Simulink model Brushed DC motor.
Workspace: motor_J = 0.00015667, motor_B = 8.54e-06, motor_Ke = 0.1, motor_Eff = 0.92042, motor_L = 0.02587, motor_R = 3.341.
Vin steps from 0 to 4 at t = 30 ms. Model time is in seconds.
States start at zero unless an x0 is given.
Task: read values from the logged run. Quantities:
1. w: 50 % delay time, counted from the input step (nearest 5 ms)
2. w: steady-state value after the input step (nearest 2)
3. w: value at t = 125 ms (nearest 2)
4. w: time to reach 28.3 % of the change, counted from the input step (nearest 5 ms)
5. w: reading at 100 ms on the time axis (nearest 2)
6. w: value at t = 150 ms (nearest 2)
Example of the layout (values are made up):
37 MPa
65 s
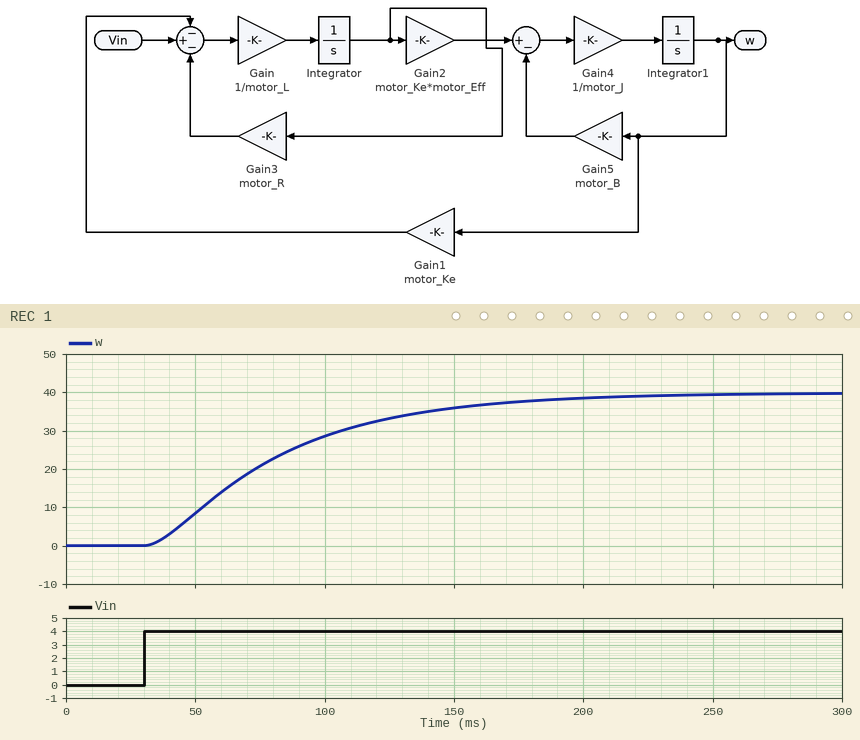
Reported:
45 ms
40
34
25 ms
28
36
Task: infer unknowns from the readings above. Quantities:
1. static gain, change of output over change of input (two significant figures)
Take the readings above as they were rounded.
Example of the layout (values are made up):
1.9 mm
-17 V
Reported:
10
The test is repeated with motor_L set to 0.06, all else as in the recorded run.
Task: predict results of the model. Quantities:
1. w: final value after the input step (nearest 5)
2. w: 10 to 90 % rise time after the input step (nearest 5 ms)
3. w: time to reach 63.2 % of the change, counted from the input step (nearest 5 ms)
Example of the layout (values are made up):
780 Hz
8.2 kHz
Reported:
40
90 ms
65 ms
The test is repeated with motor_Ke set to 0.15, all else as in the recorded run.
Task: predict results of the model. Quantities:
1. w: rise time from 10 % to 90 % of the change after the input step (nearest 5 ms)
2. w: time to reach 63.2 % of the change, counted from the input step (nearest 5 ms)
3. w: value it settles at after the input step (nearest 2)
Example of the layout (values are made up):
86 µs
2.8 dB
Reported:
40 ms
30 ms
26
